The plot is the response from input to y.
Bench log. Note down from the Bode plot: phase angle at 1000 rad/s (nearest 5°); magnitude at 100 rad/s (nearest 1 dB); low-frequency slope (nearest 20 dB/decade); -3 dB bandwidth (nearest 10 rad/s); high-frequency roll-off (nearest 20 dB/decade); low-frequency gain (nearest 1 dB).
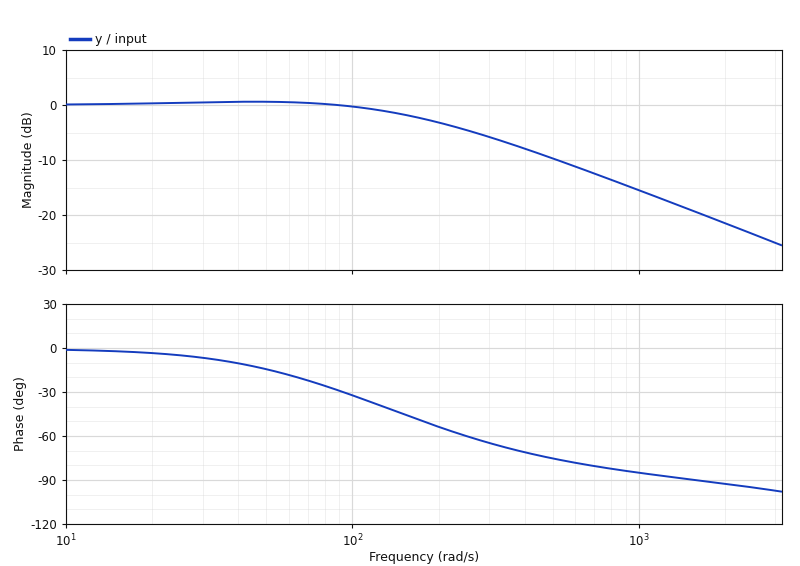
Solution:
-85°
0 dB
0 dB/decade
190 rad/s
-20 dB/decade
0 dB
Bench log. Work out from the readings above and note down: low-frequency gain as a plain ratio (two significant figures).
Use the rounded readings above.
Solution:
1.0
